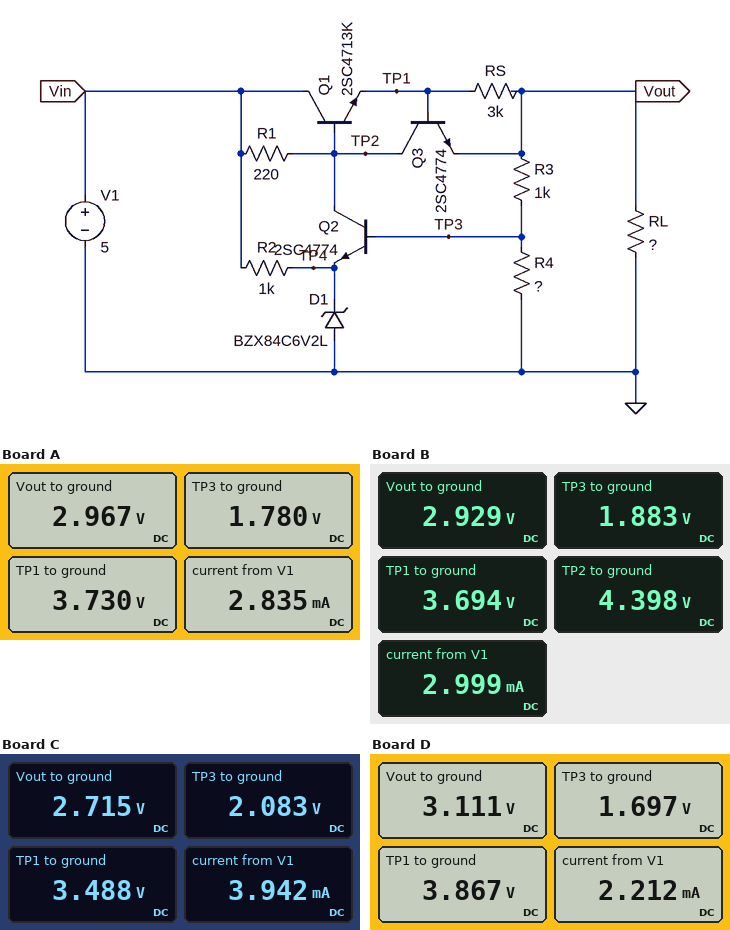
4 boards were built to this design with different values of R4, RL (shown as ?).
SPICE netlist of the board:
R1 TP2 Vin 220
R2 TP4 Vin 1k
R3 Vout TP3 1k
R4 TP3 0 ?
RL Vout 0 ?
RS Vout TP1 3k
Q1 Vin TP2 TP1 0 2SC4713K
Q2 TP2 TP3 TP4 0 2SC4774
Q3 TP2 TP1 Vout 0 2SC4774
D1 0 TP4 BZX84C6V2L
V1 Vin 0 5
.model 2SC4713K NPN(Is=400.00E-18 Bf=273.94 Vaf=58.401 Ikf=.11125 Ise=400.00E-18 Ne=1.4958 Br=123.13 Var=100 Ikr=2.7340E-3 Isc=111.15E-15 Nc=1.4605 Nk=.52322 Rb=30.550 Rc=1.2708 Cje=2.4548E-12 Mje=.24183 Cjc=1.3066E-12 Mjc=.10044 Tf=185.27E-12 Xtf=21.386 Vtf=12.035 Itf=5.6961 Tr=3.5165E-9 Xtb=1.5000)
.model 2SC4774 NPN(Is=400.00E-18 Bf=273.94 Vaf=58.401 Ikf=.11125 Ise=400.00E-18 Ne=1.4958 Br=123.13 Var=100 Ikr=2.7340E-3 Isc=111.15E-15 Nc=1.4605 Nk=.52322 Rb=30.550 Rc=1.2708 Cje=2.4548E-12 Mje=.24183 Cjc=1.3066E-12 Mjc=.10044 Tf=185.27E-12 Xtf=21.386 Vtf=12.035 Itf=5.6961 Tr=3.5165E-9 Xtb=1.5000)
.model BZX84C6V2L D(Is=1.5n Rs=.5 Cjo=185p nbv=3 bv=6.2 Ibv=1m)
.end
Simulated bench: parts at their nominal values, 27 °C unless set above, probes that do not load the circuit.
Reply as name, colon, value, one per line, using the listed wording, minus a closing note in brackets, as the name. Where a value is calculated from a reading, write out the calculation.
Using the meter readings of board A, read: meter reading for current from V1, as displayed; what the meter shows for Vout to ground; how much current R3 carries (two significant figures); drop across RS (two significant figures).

meter reading for current from V1, as displayed: 2.835 mA
what the meter shows for Vout to ground: 2.967 V
how much current R3 carries: (2.967 V - 1.78 V) / 1 kΩ = 1.2 mA
drop across RS: 3.73 V - 2.967 V = 760 mV
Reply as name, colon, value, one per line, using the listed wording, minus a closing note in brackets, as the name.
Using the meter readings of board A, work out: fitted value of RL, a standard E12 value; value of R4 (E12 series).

fitted value of RL, a standard E12 value: 1.8 kΩ
value of R4: 1.5 kΩ
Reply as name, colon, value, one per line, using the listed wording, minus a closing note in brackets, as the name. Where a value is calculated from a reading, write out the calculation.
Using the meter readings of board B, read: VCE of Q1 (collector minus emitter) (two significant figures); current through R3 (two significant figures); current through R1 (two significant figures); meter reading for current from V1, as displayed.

VCE of Q1 (collector minus emitter): 5 V - 3.694 V = 1.3 V
current through R3: (2.929 V - 1.883 V) / 1 kΩ = 1.0 mA
current through R1: (5 V - 4.398 V) / 220 Ω = 2.7 mA
meter reading for current from V1, as displayed: 2.999 mA
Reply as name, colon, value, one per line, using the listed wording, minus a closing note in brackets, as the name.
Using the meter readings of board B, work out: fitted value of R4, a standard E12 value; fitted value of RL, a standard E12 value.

fitted value of R4, a standard E12 value: 1.8 kΩ
fitted value of RL, a standard E12 value: 1.5 kΩ
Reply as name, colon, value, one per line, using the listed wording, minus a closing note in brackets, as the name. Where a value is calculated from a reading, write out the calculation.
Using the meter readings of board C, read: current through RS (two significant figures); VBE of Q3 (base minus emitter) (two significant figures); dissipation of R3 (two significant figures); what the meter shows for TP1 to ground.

current through RS: (3.488 V - 2.715 V) / 3 kΩ = 260 µA
VBE of Q3 (base minus emitter): 3.488 V - 2.715 V = 770 mV
dissipation of R3: (2.715 V - 2.083 V)^2 / 1 kΩ = 400 µW
what the meter shows for TP1 to ground: 3.488 V
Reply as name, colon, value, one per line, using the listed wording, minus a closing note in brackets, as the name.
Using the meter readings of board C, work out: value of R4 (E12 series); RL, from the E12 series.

value of R4: 3.3 kΩ
RL, from the E12 series: 820 Ω
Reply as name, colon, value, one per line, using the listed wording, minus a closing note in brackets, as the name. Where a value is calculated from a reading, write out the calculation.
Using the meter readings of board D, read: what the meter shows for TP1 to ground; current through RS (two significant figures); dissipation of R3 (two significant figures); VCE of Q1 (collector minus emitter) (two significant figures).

what the meter shows for TP1 to ground: 3.867 V
current through RS: (3.867 V - 3.111 V) / 3 kΩ = 250 µA
dissipation of R3: (3.111 V - 1.697 V)^2 / 1 kΩ = 2.0 mW
VCE of Q1 (collector minus emitter): 5 V - 3.867 V = 1.1 V
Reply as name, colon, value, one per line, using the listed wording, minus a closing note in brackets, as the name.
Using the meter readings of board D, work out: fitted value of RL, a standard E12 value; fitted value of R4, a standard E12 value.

fitted value of RL, a standard E12 value: 3.9 kΩ
fitted value of R4, a standard E12 value: 1.2 kΩ
